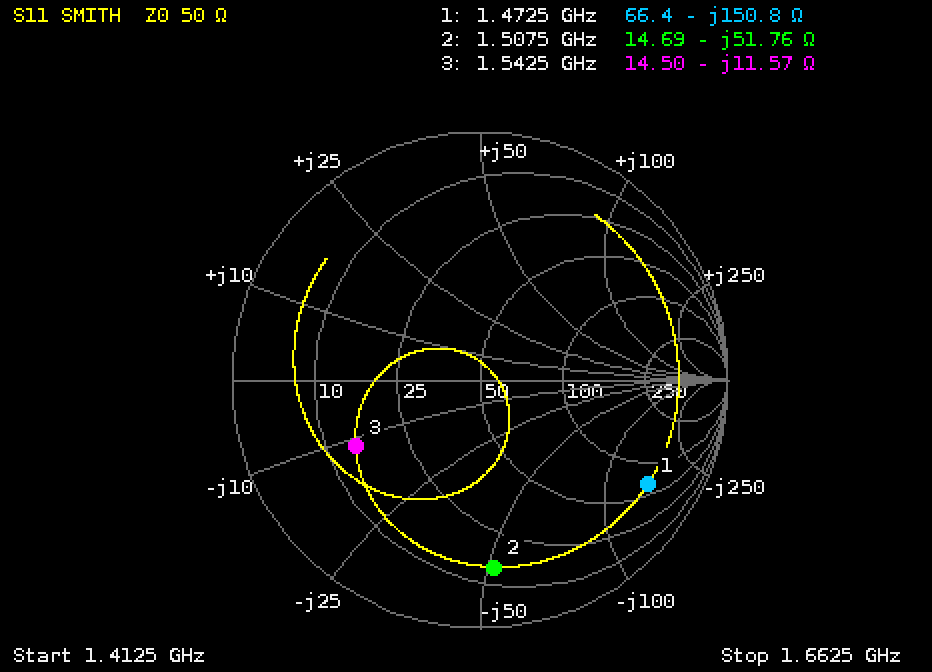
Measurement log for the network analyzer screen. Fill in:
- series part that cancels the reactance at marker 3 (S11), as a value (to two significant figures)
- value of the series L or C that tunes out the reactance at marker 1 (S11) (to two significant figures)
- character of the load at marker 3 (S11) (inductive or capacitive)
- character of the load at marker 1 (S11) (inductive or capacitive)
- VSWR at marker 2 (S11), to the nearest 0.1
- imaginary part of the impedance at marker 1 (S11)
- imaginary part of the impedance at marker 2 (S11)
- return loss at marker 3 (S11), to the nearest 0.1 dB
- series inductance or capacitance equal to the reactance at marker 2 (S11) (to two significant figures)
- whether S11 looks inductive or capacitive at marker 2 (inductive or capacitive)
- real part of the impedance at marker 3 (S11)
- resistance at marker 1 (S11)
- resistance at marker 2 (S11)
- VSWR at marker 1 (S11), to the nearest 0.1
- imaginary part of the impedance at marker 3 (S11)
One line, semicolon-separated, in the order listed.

1.2 nH; 16 nH; capacitive; capacitive; 7.2; -150.8 Ω; -51.76 Ω; 4.9 dB; 2.0 pF; capacitive; 14.50 Ω; 66.4 Ω; 14.69 Ω; 8.8; -11.57 Ω
